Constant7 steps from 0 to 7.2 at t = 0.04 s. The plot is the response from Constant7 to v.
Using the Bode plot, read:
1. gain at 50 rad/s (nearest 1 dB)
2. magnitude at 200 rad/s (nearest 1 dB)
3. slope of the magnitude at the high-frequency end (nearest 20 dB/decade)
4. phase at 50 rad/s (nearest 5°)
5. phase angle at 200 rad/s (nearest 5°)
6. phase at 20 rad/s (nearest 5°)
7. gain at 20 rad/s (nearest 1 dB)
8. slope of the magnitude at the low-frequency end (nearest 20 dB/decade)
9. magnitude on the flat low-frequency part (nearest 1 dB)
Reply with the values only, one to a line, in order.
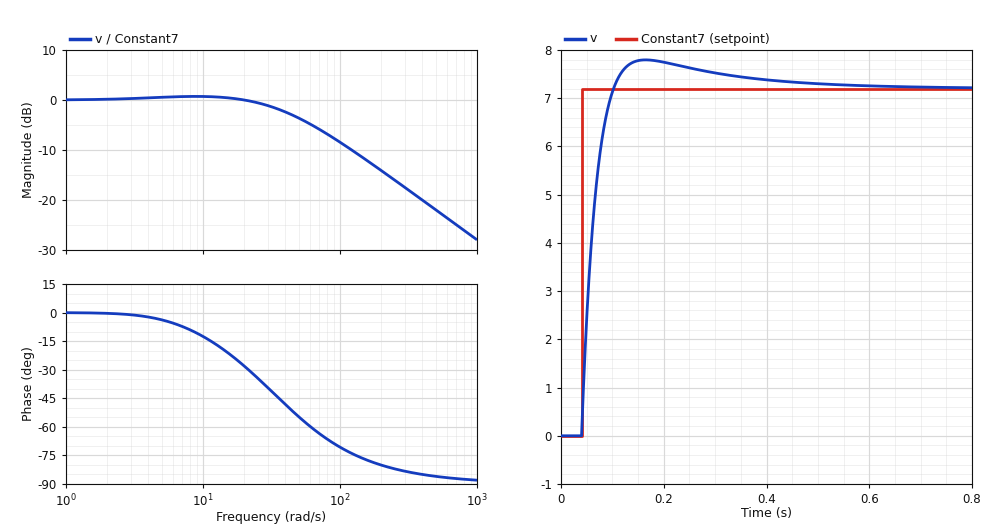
-4 dB
-14 dB
-20 dB/decade
-55°
-80°
-30°
0 dB
0 dB/decade
0 dB
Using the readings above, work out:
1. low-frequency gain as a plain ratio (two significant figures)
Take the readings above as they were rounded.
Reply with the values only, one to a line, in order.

1.0
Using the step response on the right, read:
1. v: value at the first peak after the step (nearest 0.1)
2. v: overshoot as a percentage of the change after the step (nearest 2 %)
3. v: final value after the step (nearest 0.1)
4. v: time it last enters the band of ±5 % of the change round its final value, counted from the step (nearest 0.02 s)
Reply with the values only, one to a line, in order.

7.8
8 %
7.2
0.24 s
